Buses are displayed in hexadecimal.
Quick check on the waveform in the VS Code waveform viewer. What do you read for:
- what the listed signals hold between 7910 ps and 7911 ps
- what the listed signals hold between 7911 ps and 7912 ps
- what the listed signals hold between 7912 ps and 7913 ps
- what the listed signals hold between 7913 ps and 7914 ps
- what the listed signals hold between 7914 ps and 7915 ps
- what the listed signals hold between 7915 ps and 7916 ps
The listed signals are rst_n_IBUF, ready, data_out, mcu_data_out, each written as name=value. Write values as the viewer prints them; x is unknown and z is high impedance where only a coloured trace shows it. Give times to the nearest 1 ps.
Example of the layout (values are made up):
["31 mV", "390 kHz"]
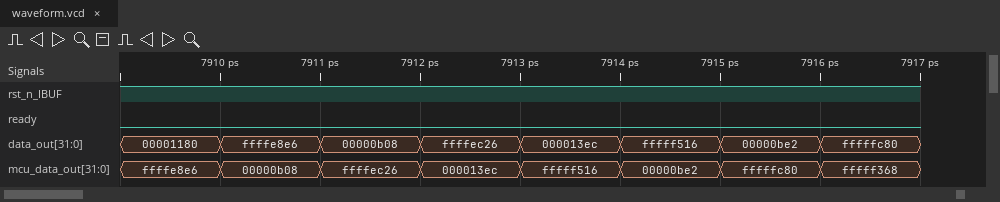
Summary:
["rst_n_IBUF=1, ready=0, data_out=ffffe8e6, mcu_data_out=00000b08", "rst_n_IBUF=1, ready=0, data_out=00000b08, mcu_data_out=ffffec26", "rst_n_IBUF=1, ready=0, data_out=ffffec26, mcu_data_out=000013ec", "rst_n_IBUF=1, ready=0, data_out=000013ec, mcu_data_out=fffff516", "rst_n_IBUF=1, ready=0, data_out=fffff516, mcu_data_out=00000be2", "rst_n_IBUF=1, ready=0, data_out=00000be2, mcu_data_out=fffffc80"]
